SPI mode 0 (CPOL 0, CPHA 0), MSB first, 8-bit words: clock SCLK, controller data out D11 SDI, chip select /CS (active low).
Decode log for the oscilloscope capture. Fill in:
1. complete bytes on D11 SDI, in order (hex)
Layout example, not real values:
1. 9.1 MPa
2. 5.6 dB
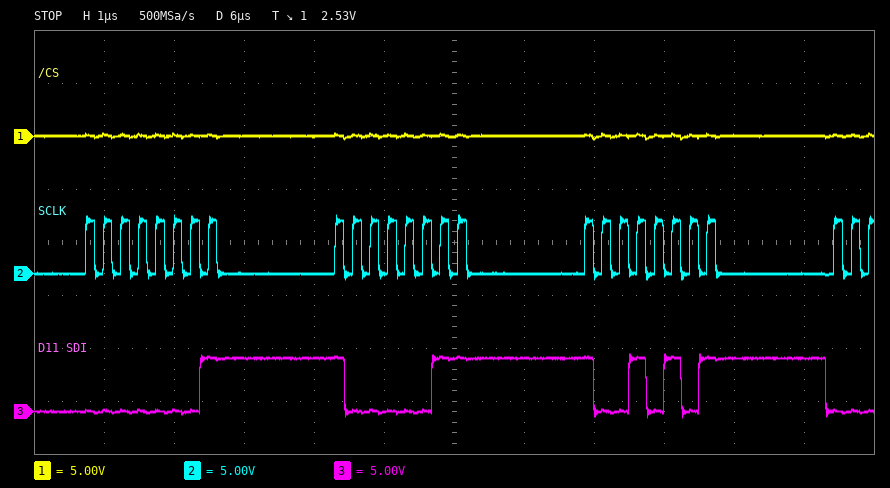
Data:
1. 01 83 95
